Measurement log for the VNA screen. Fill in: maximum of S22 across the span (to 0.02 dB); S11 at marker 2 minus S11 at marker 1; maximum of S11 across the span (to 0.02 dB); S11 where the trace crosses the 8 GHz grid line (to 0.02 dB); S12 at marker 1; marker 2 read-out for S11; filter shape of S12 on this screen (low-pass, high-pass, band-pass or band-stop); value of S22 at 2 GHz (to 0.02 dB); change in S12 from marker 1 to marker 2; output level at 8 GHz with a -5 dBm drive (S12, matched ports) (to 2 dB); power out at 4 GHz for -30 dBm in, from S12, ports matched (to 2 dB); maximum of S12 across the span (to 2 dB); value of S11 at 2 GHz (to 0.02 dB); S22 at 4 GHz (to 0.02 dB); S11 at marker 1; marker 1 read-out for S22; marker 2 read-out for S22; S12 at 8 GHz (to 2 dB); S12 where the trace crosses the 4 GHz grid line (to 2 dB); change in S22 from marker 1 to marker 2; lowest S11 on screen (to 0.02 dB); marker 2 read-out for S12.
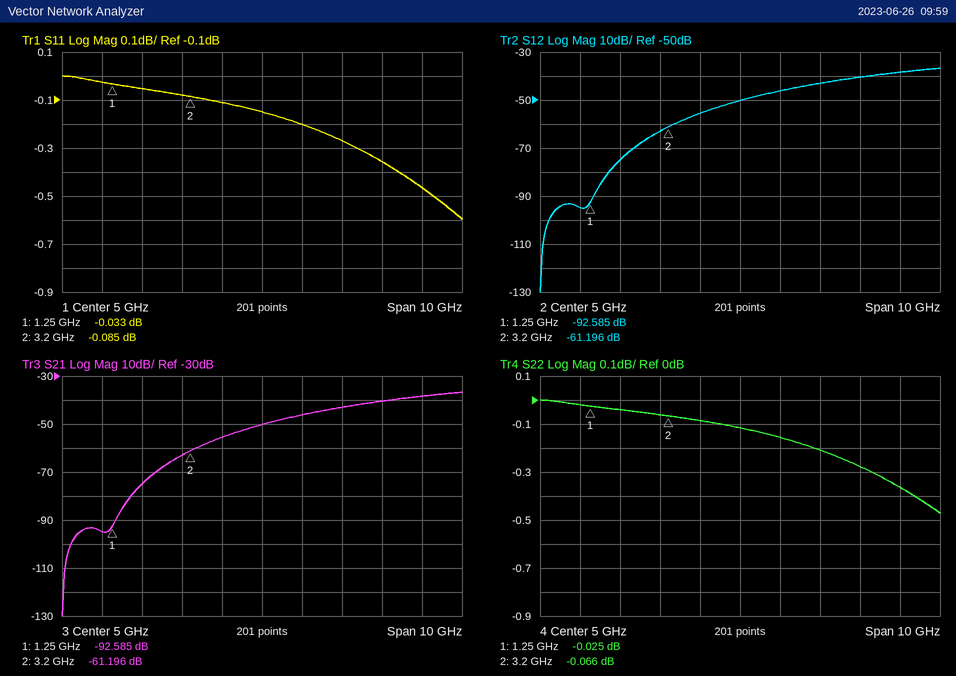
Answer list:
0.00 dB
-0.052 dB
0.00 dB
-0.36 dB
-92.585 dB
-0.085 dB
high-pass
-0.04 dB
31.389 dB
-46 dBm
-86 dBm
-36 dB
-0.06 dB
-0.08 dB
-0.033 dB
-0.025 dB
-0.066 dB
-40 dB
-56 dB
-0.041 dB
-0.60 dB
-61.196 dB
